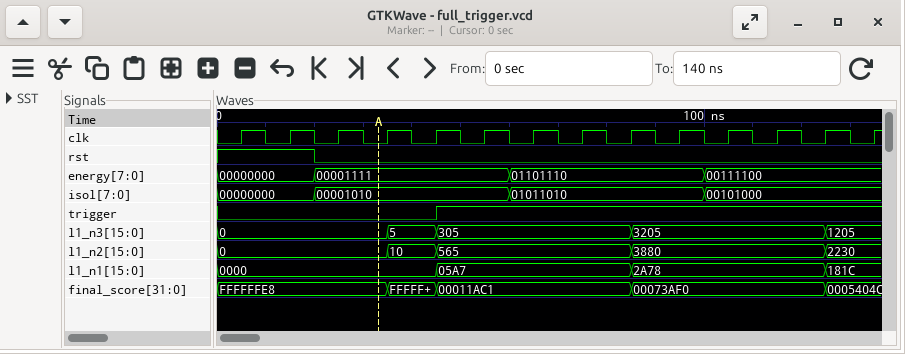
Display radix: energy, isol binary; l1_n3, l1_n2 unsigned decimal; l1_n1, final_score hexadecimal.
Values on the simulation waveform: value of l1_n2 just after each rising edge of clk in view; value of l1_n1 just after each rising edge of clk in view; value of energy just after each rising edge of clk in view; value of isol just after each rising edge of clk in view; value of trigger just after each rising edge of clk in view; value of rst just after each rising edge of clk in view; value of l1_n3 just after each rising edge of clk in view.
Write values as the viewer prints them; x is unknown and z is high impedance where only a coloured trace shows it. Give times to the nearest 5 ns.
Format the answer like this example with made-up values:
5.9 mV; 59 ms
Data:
0, 0, 0, 10, 565, 565, 565, 565, 3880, 3880, 3880, 3880, 2230, 2230; 0000, 0000, 0000, 0000, 05A7, 05A7, 05A7, 05A7, 2A78, 2A78, 2A78, 2A78, 181C, 181C; 00000000, 00000000, 00001111, 00001111, 00001111, 00001111, 01101110, 01101110, 01101110, 01101110, 00111100, 00111100, 00111100, 00111100; 00000000, 00000000, 00001010, 00001010, 00001010, 00001010, 01011010, 01011010, 01011010, 01011010, 00101000, 00101000, 00101000, 00101000; 0 0 0 0 1 1 1 1 1 1 1 1 1 1; 1 1 0 0 0 0 0 0 0 0 0 0 0 0; 0, 0, 0, 5, 305, 305, 305, 305, 3205, 3205, 3205, 3205, 1205, 1205
